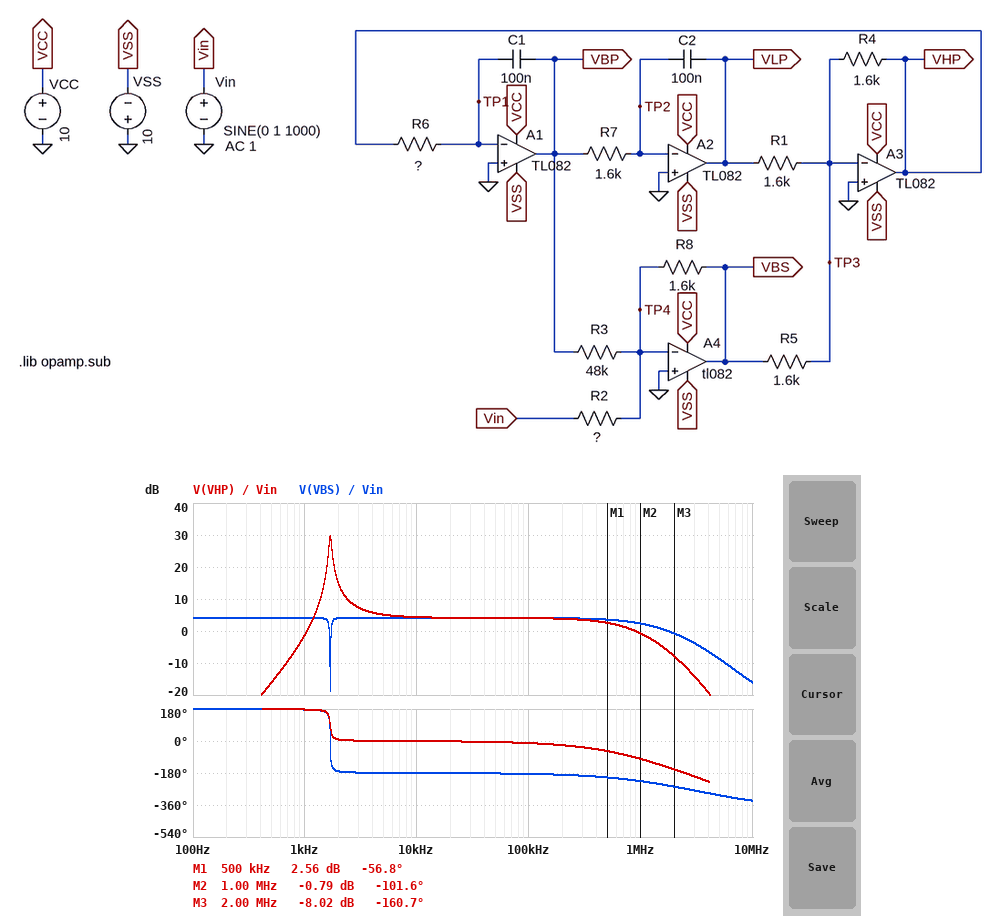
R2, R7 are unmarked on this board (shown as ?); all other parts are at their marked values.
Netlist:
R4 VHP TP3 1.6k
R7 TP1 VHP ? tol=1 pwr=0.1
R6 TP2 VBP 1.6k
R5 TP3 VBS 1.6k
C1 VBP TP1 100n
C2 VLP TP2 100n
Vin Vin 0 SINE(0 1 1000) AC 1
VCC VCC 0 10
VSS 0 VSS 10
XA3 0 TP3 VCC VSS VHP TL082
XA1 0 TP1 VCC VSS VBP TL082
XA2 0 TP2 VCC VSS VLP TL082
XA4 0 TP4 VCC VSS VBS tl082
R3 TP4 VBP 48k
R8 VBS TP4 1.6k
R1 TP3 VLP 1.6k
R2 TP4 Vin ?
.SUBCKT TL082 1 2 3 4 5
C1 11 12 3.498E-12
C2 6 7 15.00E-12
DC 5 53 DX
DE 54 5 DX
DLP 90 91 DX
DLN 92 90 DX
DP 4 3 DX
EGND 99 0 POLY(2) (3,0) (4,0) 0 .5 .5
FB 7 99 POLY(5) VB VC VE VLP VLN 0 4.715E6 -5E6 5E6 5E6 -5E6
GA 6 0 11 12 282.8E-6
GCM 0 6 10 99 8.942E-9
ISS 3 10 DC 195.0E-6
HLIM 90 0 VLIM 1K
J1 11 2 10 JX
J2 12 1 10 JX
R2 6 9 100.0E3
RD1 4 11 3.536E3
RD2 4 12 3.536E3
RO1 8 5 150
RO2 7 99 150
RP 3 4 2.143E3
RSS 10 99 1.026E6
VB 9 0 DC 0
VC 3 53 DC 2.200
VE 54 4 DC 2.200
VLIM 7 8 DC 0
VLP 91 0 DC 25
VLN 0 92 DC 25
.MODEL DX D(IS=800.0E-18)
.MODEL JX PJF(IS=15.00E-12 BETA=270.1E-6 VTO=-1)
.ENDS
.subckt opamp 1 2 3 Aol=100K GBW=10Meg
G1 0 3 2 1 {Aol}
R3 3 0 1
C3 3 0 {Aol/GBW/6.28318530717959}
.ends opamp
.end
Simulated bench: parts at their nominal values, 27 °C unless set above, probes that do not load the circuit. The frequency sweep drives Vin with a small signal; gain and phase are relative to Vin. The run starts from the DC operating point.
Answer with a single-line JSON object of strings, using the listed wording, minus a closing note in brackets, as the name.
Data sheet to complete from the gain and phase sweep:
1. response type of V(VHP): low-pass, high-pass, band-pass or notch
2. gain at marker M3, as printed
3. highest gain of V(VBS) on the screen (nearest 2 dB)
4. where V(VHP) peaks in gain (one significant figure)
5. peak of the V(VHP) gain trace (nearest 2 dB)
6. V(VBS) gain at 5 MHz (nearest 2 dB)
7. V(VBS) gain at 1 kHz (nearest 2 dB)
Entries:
{"response type of V(VHP): low-pass, high-pass, band-pass or notch": "band-pass", "gain at marker M3, as printed": "-8.02 dB", "highest gain of V(VBS) on the screen": "4 dB", "where V(VHP) peaks in gain": "2 kHz", "peak of the V(VHP) gain trace": "30 dB", "V(VBS) gain at 5 MHz": "-8 dB", "V(VBS) gain at 1 kHz": "4 dB"}
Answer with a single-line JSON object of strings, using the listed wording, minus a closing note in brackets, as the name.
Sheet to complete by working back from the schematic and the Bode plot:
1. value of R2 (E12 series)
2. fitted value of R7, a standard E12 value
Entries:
{"value of R2": "1 kΩ", "fitted value of R7, a standard E12 value": "560 Ω"}
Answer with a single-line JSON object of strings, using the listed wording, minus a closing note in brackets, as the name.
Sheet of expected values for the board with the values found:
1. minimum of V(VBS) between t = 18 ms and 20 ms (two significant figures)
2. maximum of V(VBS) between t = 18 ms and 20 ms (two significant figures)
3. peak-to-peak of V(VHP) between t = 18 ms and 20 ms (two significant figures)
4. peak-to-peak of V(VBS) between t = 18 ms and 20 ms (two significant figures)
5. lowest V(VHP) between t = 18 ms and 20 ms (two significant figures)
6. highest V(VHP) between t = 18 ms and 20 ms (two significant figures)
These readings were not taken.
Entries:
{"minimum of V(VBS) between t = 18 ms and 20 ms": "-1.6 V", "maximum of V(VBS) between t = 18 ms and 20 ms": "1.6 V", "peak-to-peak of V(VHP) between t = 18 ms and 20 ms": "1.8 V", "peak-to-peak of V(VBS) between t = 18 ms and 20 ms": "3.2 V", "lowest V(VHP) between t = 18 ms and 20 ms": "-880 mV", "highest V(VHP) between t = 18 ms and 20 ms": "880 mV"}
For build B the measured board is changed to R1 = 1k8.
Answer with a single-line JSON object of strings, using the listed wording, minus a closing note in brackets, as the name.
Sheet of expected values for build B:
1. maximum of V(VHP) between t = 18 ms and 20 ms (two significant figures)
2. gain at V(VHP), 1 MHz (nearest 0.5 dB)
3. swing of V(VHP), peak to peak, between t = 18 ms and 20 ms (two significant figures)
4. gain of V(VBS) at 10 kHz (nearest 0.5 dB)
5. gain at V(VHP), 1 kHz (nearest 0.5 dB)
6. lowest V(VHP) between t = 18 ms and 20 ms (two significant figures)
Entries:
{"maximum of V(VHP) between t = 18 ms and 20 ms": "1.1 V", "gain at V(VHP), 1 MHz": "-0.5 dB", "swing of V(VHP), peak to peak, between t = 18 ms and 20 ms": "2.1 V", "gain of V(VBS) at 10 kHz": "4.0 dB", "gain at V(VHP), 1 kHz": "0.5 dB", "lowest V(VHP) between t = 18 ms and 20 ms": "-1.1 V"}
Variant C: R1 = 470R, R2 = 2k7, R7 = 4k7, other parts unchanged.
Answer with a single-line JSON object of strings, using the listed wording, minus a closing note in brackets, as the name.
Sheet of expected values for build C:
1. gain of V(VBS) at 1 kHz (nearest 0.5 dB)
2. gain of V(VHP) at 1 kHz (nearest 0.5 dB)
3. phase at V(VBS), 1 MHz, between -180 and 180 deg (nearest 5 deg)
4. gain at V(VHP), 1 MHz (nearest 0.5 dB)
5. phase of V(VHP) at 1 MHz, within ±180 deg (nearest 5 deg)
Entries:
{"gain of V(VBS) at 1 kHz": "-4.5 dB", "gain of V(VHP) at 1 kHz": "12.0 dB", "phase at V(VBS), 1 MHz, between -180 and 180 deg": "150 deg", "gain at V(VHP), 1 MHz": "-10.5 dB", "phase of V(VHP) at 1 MHz, within ±180 deg": "-95 deg"}
